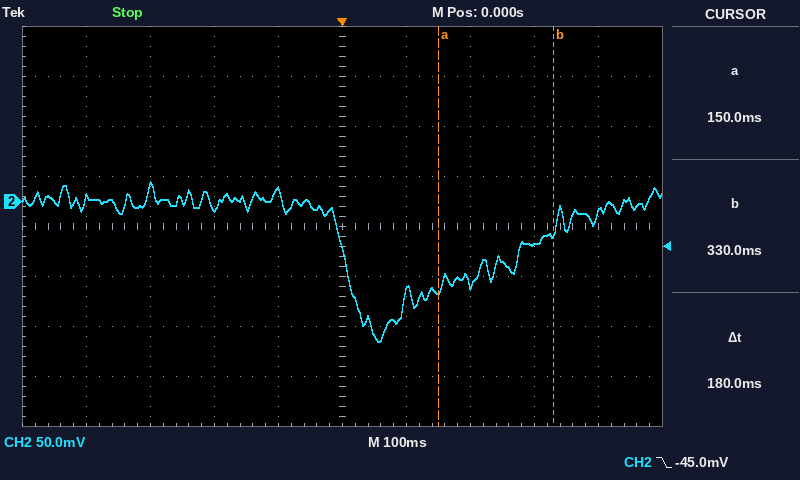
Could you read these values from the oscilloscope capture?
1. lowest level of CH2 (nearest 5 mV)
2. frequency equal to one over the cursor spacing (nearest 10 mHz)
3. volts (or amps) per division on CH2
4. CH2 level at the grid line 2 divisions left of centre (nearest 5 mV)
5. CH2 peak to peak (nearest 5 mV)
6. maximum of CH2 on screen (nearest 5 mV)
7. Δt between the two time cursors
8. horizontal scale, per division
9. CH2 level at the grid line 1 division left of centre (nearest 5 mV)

-140 mV
5.56 Hz
50 mV
-5 mV
160 mV
20 mV
180 ms
100 ms
10 mV
